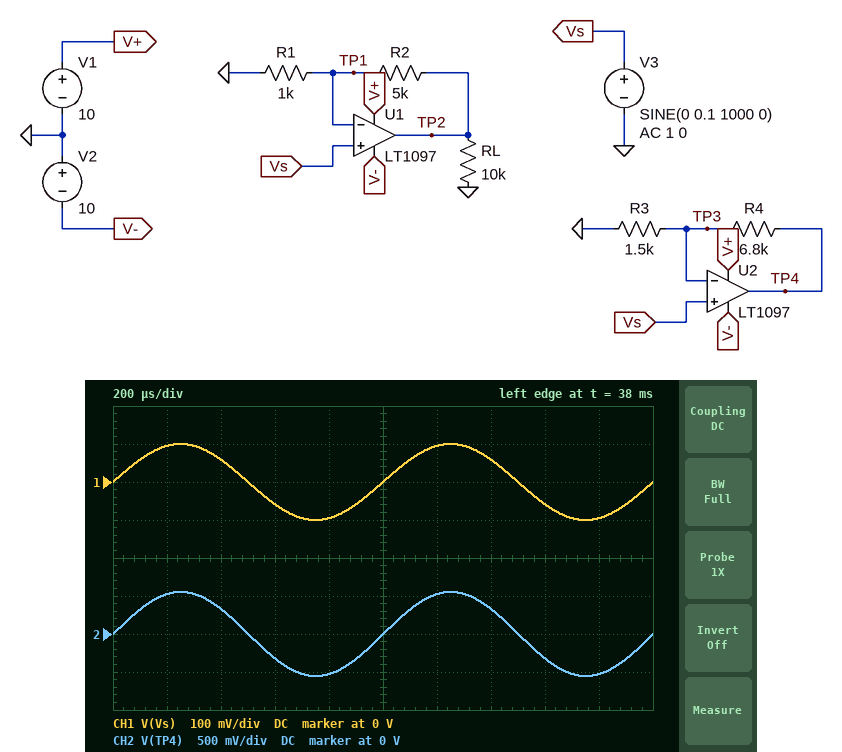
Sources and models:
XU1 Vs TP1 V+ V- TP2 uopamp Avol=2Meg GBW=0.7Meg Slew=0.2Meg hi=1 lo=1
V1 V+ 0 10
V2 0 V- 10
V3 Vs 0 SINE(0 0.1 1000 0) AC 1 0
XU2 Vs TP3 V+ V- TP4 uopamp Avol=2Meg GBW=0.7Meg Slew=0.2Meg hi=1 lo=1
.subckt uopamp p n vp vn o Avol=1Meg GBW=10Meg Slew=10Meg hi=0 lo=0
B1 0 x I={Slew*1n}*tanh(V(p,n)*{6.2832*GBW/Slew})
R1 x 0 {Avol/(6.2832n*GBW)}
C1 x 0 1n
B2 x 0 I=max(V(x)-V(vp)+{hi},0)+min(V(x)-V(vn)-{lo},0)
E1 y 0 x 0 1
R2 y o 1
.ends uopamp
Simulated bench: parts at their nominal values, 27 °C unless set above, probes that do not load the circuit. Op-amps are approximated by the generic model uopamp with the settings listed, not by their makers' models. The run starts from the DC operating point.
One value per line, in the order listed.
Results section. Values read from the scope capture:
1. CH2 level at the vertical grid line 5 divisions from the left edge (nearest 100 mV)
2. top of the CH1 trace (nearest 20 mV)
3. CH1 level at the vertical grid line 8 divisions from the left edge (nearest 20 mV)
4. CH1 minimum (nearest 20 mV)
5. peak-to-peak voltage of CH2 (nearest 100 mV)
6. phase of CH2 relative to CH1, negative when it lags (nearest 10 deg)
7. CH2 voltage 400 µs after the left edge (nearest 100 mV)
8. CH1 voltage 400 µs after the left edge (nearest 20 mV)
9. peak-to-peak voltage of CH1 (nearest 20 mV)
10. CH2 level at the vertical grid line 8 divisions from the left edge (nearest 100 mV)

0 V
100 mV
-60 mV
-100 mV
1.1 V
0 deg
300 mV
60 mV
200 mV
-300 mV
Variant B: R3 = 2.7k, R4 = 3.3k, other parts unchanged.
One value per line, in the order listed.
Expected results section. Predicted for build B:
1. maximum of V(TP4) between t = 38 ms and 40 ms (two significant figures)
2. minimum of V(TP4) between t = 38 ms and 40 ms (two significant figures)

220 mV
-220 mV
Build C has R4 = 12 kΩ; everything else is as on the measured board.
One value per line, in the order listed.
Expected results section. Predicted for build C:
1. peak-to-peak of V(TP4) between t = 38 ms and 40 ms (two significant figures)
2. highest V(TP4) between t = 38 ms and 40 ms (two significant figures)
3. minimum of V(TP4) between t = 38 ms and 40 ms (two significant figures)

1.8 V
900 mV
-900 mV
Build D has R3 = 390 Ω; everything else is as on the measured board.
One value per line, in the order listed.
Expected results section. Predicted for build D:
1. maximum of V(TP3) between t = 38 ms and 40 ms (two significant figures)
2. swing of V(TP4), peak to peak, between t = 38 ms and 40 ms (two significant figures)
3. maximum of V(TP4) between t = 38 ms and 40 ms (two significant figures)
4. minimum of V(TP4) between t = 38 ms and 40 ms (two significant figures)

100 mV
3.7 V
1.8 V
-1.8 V
